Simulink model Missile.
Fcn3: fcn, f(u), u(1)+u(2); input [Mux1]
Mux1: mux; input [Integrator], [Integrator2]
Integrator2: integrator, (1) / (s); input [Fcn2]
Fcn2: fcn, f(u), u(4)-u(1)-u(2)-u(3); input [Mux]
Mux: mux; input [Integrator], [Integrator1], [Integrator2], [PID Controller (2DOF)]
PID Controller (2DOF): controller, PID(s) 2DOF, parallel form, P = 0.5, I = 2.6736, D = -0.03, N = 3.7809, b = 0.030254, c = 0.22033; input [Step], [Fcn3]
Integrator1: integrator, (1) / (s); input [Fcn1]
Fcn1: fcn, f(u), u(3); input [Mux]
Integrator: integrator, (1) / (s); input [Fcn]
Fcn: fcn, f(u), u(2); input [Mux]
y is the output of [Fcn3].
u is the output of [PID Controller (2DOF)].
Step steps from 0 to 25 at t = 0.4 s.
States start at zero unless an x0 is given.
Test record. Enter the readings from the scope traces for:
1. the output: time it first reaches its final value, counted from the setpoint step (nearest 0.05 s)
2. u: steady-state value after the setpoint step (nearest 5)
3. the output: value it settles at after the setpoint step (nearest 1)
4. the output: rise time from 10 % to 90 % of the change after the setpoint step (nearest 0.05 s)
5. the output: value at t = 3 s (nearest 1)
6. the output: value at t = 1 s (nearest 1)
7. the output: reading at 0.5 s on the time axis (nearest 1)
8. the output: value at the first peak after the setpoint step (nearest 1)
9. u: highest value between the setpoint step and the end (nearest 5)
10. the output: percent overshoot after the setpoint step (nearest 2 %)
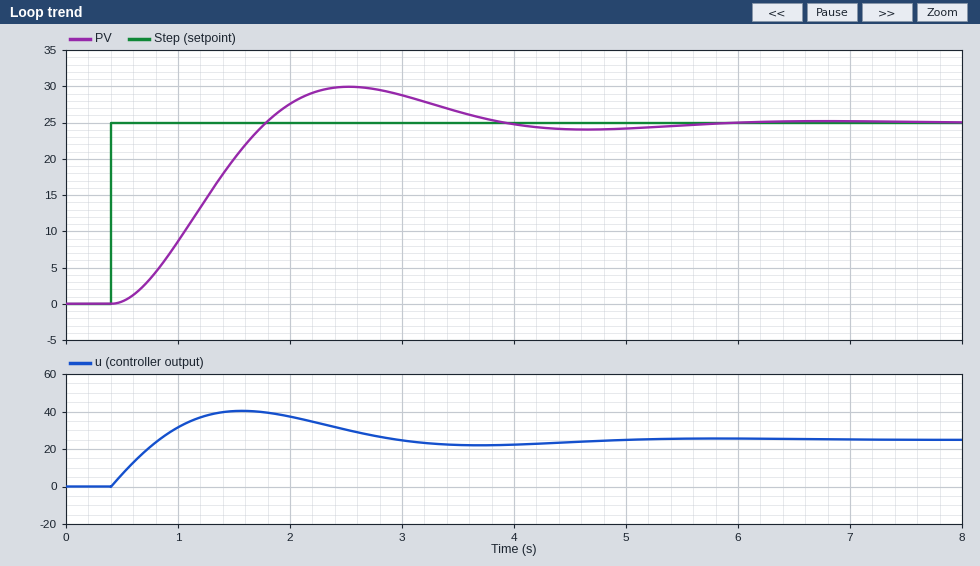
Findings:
1.40 s
25
25
0.95 s
29
9
0
30
40
20 %
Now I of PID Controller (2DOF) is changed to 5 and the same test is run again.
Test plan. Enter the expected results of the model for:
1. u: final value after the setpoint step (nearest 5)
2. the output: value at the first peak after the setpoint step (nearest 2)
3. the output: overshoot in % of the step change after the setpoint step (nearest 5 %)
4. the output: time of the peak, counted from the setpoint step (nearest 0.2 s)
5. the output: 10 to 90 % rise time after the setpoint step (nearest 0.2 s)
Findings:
25
34
35 %
1.4 s
0.6 s
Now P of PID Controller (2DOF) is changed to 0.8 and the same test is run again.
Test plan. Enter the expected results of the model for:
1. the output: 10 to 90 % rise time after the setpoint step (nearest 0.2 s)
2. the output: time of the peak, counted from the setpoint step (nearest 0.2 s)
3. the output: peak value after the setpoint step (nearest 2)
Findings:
1.0 s
2.2 s
28
